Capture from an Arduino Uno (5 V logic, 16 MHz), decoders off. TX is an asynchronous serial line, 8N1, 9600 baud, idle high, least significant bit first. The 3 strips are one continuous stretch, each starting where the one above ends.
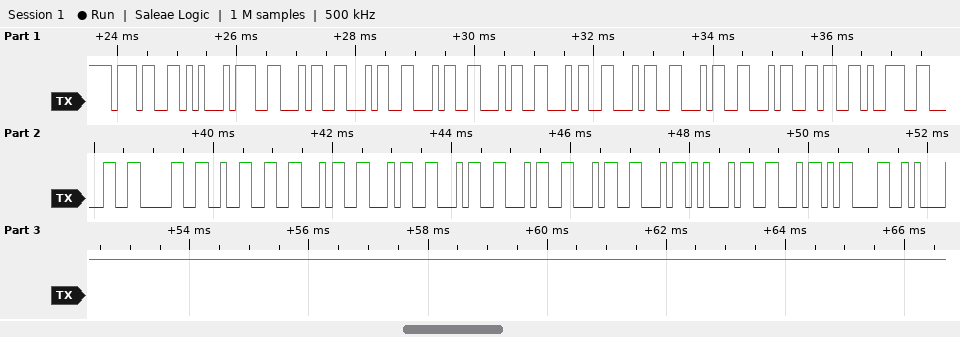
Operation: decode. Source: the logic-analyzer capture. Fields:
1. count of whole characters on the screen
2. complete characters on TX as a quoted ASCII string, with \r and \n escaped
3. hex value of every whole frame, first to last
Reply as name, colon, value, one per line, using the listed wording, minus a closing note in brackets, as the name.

count of whole characters on the screen: 25
complete characters on TX as a quoted ASCII string, with \r and \n escaped: "7EFFFFFFFF69002FFFFFFEF\r\n"
hex value of every whole frame, first to last: 37 45 46 46 46 46 46 46 46 46 36 39 30 30 32 46 46 46 46 46 46 45 46 0D 0A
